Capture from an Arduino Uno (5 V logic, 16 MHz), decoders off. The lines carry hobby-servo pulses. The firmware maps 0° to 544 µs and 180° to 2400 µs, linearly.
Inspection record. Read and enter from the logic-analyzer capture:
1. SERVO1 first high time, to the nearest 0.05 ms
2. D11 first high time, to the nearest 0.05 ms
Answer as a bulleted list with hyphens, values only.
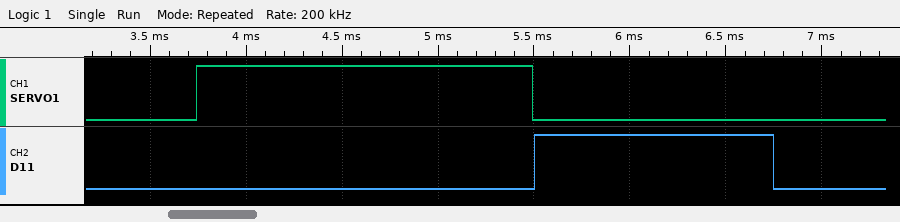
- 1.75 ms
- 1.25 ms
